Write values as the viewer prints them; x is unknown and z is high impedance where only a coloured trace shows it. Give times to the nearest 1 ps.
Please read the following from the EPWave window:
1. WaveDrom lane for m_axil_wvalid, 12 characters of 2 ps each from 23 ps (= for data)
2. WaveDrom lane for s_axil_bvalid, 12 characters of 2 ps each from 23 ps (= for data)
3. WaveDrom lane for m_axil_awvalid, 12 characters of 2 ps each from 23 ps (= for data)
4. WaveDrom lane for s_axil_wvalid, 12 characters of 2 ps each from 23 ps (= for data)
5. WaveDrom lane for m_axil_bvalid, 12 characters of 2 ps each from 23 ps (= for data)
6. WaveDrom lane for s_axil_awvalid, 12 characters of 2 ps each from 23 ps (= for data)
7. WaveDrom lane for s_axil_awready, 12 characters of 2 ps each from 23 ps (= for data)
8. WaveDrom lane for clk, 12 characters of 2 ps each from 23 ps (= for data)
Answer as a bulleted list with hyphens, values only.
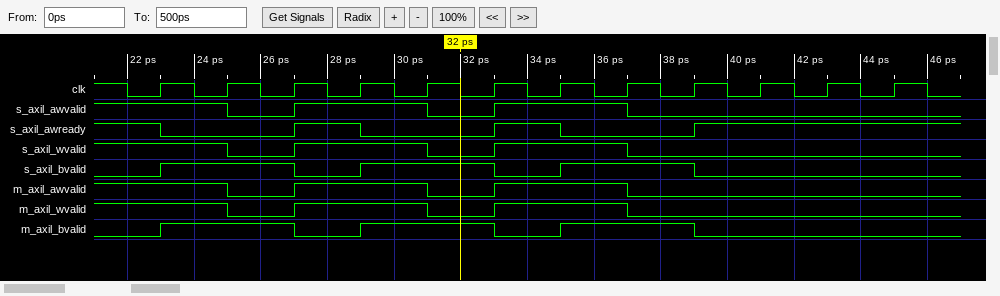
- {name: 'm_axil_wvalid', wave: '101.01.0....'}
- {name: 's_axil_bvalid', wave: '1.01.01.0...'}
- {name: 'm_axil_awvalid', wave: '101.01.0....'}
- {name: 's_axil_wvalid', wave: '101.01.0....'}
- {name: 'm_axil_bvalid', wave: '1.01.01.0...'}
- {name: 's_axil_awvalid', wave: '101.01.0....'}
- {name: 's_axil_awready', wave: '0.10.10.1...'}
- {name: 'clk', wave: 'p...........'}
